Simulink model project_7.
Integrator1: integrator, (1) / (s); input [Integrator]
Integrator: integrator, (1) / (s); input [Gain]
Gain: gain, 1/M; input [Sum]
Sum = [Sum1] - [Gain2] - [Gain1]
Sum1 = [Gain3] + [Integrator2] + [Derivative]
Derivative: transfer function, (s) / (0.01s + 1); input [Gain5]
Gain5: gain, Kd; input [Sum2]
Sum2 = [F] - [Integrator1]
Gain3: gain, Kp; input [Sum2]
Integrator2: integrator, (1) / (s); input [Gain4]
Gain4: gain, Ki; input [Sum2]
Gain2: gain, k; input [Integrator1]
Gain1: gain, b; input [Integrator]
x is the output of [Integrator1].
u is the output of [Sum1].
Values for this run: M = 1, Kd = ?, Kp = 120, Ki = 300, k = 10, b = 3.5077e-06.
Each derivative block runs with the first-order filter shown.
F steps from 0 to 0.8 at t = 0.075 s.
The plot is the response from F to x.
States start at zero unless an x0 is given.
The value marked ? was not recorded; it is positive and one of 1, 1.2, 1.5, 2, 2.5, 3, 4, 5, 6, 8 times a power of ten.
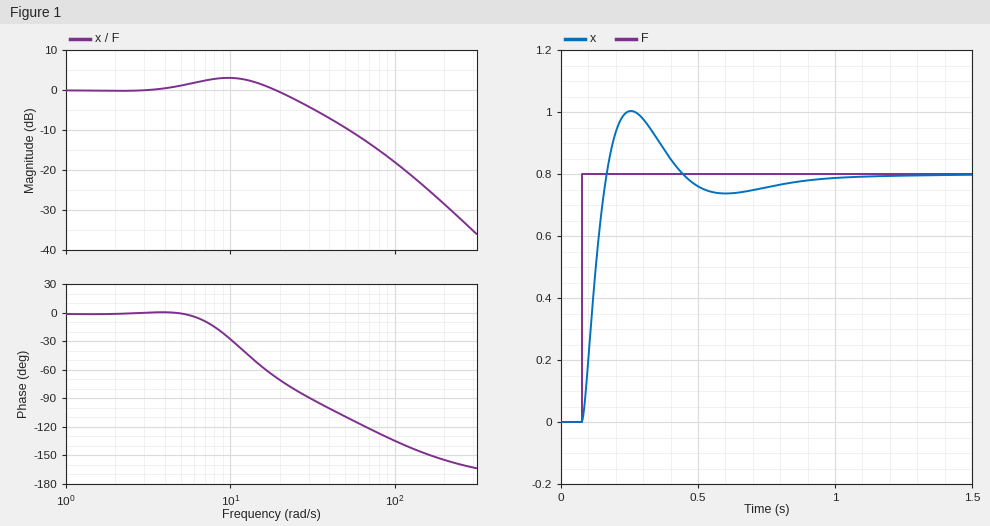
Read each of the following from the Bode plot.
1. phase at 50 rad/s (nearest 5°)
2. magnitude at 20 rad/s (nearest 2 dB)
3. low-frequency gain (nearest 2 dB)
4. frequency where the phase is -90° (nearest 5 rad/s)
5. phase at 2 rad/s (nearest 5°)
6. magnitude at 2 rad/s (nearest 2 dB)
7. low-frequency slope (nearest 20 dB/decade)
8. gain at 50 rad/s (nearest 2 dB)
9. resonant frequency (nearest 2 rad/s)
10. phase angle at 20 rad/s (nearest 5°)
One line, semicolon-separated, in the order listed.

-110°; 0 dB; 0 dB; 30 rad/s; 0°; 0 dB; 0 dB/decade; -10 dB; 10 rad/s; -70°
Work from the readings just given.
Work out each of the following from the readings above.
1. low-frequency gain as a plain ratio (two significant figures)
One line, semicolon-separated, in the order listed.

1.0
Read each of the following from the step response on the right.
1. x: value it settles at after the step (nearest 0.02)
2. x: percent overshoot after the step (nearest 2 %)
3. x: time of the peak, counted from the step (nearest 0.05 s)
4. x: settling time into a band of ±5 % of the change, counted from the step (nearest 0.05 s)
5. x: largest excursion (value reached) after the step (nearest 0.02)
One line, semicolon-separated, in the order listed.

0.80; 26 %; 0.20 s; 0.70 s; 1.00
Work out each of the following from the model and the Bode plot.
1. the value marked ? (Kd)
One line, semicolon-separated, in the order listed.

15
